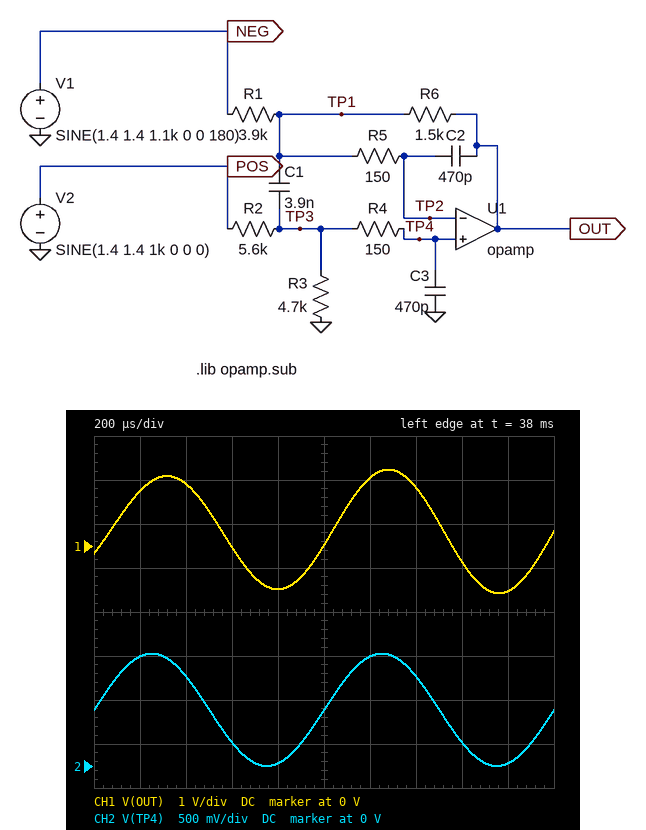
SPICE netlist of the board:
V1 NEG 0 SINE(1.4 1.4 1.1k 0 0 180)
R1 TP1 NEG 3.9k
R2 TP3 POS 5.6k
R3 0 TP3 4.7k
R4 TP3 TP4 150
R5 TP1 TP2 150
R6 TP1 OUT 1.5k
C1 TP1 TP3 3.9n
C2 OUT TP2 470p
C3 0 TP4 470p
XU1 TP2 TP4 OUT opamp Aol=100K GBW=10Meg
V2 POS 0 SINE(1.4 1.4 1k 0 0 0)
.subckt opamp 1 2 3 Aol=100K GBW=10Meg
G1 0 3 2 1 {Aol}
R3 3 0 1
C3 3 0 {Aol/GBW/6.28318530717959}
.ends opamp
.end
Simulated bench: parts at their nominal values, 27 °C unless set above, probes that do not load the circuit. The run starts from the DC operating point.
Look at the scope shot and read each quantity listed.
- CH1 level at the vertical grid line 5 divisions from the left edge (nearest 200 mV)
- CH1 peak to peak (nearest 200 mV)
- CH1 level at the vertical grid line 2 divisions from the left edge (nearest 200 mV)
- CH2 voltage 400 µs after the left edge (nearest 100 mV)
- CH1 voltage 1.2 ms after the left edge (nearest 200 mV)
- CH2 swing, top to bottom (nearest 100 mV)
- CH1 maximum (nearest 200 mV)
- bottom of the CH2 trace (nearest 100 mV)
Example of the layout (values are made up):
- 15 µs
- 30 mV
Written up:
- 0 V
- 2.8 V
- 1.4 V
- 1.0 V
- 1.6 V
- 1.3 V
- 1.8 V
- 0 V
